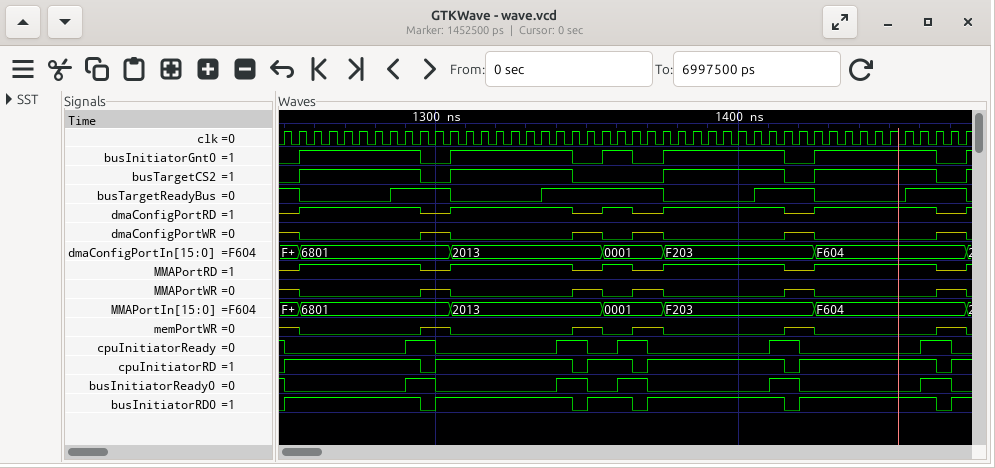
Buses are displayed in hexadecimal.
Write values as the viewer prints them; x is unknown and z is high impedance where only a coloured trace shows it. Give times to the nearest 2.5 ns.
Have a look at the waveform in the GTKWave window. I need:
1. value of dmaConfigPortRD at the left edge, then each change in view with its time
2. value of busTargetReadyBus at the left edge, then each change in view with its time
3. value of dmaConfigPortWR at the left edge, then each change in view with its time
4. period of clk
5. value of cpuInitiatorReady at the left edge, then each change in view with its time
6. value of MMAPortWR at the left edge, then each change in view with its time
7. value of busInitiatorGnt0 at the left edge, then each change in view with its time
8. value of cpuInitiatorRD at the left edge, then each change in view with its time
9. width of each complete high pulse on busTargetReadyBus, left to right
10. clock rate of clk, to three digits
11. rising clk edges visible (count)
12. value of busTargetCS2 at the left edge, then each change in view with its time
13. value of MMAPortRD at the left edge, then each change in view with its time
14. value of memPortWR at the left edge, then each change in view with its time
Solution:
z, 1 at 1255 ns, z at 1295 ns, 1 at 1305 ns, z at 1345 ns, 1 at 1355 ns, z at 1365 ns, 1 at 1375 ns, z at 1415 ns, 1 at 1425 ns, z at 1465 ns, 1 at 1475 ns
1, 0 at 1255 ns, 1 at 1285 ns, 0 at 1305 ns, 1 at 1335 ns, 0 at 1375 ns, 1 at 1405 ns, 0 at 1425 ns, 1 at 1455 ns, 0 at 1475 ns
z, 0 at 1255 ns, z at 1295 ns, 0 at 1305 ns, z at 1345 ns, 0 at 1355 ns, z at 1365 ns, 0 at 1375 ns, z at 1415 ns, 0 at 1425 ns, z at 1465 ns, 0 at 1475 ns
5 ns
1, 0 at 1250 ns, 1 at 1290 ns, 0 at 1300 ns, 1 at 1340 ns, 0 at 1350 ns, 1 at 1360 ns, 0 at 1370 ns, 1 at 1410 ns, 0 at 1420 ns, 1 at 1460 ns, 0 at 1470 ns
z, 0 at 1255 ns, z at 1295 ns, 0 at 1305 ns, z at 1345 ns, 0 at 1355 ns, z at 1365 ns, 0 at 1375 ns, z at 1415 ns, 0 at 1425 ns, z at 1465 ns, 0 at 1475 ns
0, 1 at 1255 ns, 0 at 1295 ns, 1 at 1305 ns, 0 at 1345 ns, 1 at 1355 ns, 0 at 1365 ns, 1 at 1375 ns, 0 at 1415 ns, 1 at 1425 ns, 0 at 1465 ns, 1 at 1475 ns
0, 1 at 1250 ns, 0 at 1295 ns, 1 at 1300 ns, 0 at 1345 ns, 1 at 1350 ns, 0 at 1365 ns, 1 at 1370 ns, 0 at 1415 ns, 1 at 1420 ns, 0 at 1465 ns, 1 at 1470 ns
20 ns, 40 ns, 20 ns, 20 ns
200 MHz
46
0, 1 at 1255 ns, 0 at 1295 ns, 1 at 1305 ns, 0 at 1345 ns, 1 at 1375 ns, 0 at 1415 ns, 1 at 1425 ns, 0 at 1465 ns, 1 at 1475 ns
z, 1 at 1255 ns, z at 1295 ns, 1 at 1305 ns, z at 1345 ns, 1 at 1355 ns, z at 1365 ns, 1 at 1375 ns, z at 1415 ns, 1 at 1425 ns, z at 1465 ns, 1 at 1475 ns
z, 0 at 1255 ns, z at 1295 ns, 0 at 1305 ns, z at 1345 ns, 0 at 1355 ns, z at 1365 ns, 0 at 1375 ns, z at 1415 ns, 0 at 1425 ns, z at 1465 ns, 0 at 1475 ns
